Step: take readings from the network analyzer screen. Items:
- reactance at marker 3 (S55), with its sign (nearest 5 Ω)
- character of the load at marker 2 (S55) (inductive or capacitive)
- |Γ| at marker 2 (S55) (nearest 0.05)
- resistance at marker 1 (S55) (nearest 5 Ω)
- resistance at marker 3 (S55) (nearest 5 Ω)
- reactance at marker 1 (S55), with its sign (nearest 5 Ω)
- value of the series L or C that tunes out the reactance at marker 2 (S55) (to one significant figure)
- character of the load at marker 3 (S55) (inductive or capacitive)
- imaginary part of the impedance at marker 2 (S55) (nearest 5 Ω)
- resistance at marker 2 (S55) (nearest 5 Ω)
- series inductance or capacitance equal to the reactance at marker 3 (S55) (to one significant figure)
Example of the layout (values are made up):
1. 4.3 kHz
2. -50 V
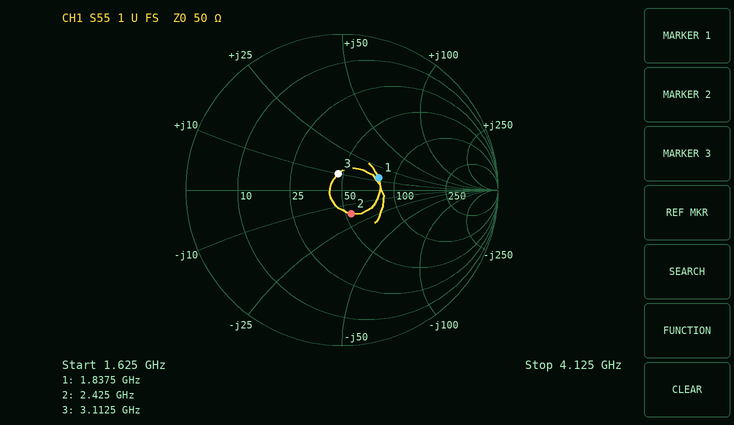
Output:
1. +10 Ω
2. capacitive
3. 0.15
4. 80 Ω
5. 45 Ω
6. +15 Ω
7. 1 nH
8. inductive
9. -15 Ω
10. 55 Ω
11. 500 pH
